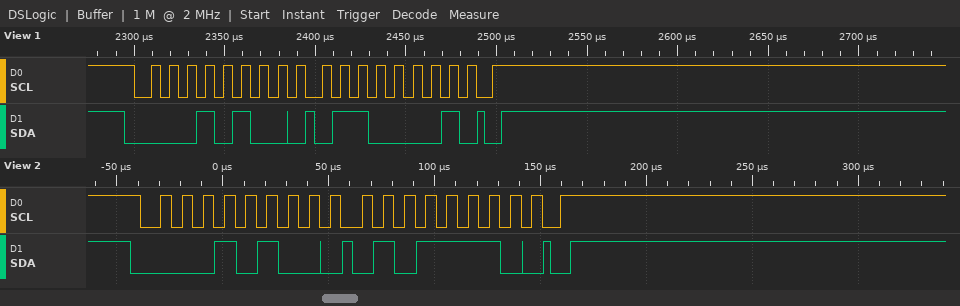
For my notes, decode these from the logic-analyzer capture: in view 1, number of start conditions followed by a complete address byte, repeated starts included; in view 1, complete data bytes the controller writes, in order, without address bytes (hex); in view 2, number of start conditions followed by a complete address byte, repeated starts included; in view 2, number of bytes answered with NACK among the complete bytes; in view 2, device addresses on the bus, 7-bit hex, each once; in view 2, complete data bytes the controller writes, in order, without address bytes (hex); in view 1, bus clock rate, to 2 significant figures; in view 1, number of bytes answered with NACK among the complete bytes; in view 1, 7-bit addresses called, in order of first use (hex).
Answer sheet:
1
61
1
0
0x0A
5E
100 kHz
0
0x0A
